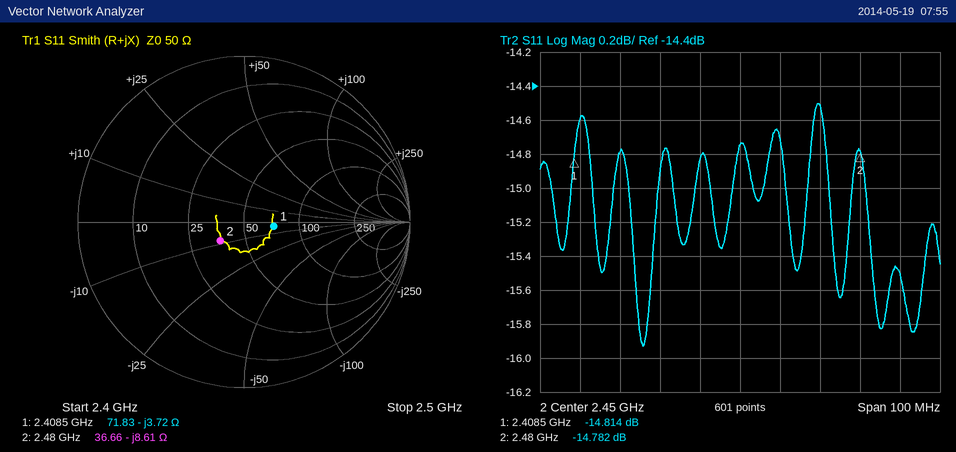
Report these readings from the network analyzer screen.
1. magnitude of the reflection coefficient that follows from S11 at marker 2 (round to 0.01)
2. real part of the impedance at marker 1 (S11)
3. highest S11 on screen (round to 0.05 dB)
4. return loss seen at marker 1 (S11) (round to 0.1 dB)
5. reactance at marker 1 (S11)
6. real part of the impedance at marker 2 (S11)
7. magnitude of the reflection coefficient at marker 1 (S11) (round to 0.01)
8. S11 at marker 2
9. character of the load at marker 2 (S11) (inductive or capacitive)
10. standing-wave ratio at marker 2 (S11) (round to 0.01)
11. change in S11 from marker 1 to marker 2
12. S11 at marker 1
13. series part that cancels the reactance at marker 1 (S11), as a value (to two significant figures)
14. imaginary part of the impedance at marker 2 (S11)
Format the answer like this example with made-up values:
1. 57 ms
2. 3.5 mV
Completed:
1. 0.18
2. 71.83 Ω
3. -14.50 dB
4. 14.8 dB
5. -3.72 Ω
6. 36.66 Ω
7. 0.18
8. -14.782 dB
9. capacitive
10. 1.45
11. 0.032 dB
12. -14.814 dB
13. 250 pH
14. -8.61 Ω
